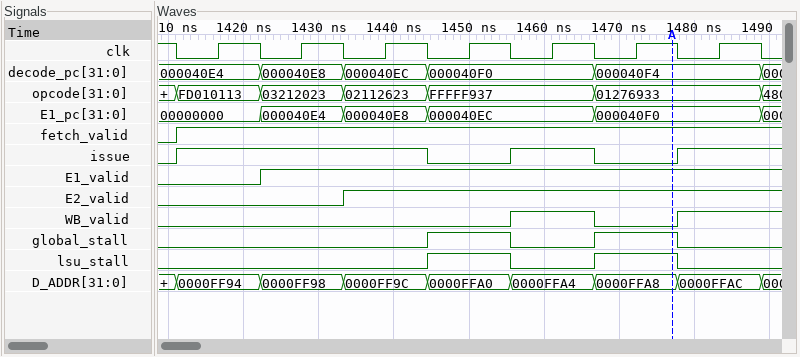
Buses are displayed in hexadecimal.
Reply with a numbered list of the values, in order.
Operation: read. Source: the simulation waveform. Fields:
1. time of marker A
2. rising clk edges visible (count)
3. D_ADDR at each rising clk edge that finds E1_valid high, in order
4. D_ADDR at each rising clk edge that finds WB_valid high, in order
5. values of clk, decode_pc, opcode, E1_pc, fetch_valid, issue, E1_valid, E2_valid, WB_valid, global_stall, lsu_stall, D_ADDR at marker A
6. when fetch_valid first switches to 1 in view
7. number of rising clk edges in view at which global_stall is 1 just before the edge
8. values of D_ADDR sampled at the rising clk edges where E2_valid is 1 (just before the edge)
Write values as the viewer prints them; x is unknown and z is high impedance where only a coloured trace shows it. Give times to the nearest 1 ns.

1. 1477 ns
2. 7
3. 0000FF98, 0000FF9C, 0000FFA0, 0000FFA4, 0000FFA8, 0000FFAC
4. 0000FFA4, 0000FFAC
5. clk=1, decode_pc=000040F4, opcode=01276933, E1_pc=000040F0, fetch_valid=1, issue=0, E1_valid=1, E2_valid=1, WB_valid=0, global_stall=1, lsu_stall=1, D_ADDR=0000FFA8
6. 1411 ns
7. 2
8. 0000FF9C, 0000FFA0, 0000FFA4, 0000FFA8, 0000FFAC
